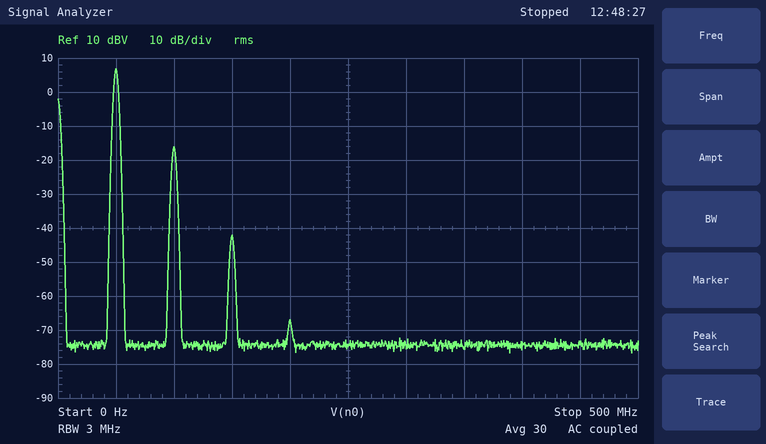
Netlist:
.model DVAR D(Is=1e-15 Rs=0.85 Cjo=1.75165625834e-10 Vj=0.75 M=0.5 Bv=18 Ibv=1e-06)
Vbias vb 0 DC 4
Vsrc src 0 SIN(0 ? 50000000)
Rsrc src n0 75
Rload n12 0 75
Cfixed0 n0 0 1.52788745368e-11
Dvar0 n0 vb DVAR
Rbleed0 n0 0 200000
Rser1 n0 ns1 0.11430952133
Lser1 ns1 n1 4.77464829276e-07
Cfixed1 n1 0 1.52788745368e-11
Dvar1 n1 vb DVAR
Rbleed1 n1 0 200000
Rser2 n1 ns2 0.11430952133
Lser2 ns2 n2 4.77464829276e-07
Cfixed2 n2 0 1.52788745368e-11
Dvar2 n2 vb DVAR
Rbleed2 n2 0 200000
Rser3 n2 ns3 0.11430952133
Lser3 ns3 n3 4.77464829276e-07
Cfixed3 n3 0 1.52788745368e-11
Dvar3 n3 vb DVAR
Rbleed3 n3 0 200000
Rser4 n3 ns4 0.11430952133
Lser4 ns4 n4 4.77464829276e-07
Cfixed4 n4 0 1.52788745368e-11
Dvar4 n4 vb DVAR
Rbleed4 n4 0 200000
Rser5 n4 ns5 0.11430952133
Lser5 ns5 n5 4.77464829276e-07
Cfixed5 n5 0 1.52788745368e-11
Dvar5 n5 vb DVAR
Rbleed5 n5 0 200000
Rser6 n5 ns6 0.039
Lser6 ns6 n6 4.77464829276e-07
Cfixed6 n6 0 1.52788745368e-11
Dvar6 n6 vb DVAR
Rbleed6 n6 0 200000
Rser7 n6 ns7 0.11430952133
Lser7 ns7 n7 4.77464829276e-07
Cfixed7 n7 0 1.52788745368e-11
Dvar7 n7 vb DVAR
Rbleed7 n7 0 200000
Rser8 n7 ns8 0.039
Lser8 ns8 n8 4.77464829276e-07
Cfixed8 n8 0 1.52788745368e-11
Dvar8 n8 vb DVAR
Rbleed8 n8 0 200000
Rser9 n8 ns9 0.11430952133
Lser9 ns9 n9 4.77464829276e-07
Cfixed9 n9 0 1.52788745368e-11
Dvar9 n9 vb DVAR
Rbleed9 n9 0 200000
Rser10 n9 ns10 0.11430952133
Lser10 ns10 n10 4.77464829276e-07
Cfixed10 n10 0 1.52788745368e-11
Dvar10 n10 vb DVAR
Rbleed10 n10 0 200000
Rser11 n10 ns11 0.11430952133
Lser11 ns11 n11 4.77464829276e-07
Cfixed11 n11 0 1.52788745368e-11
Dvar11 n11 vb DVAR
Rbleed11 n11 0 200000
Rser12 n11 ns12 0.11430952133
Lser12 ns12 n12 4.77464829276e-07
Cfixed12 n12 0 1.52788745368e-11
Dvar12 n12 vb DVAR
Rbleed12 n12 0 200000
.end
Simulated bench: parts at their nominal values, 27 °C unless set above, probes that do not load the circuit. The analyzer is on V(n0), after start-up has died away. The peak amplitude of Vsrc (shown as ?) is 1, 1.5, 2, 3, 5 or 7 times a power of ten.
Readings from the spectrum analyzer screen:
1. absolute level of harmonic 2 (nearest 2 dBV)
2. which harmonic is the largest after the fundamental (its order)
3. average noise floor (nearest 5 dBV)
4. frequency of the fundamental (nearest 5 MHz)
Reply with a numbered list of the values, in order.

1. -16 dBV
2. 2
3. -75 dBV
4. 50 MHz
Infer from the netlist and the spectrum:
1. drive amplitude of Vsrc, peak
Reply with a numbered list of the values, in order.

1. 5 V
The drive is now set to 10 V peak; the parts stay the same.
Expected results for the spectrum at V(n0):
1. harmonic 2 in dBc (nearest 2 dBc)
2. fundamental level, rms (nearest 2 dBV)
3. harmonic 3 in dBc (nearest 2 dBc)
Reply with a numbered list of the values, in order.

1. -16 dBc
2. 12 dBV
3. -36 dBc
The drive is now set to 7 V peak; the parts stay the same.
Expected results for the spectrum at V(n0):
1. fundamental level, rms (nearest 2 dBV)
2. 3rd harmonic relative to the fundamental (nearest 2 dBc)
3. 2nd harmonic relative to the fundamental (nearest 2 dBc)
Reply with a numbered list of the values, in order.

1. 10 dBV
2. -42 dBc
3. -20 dBc
